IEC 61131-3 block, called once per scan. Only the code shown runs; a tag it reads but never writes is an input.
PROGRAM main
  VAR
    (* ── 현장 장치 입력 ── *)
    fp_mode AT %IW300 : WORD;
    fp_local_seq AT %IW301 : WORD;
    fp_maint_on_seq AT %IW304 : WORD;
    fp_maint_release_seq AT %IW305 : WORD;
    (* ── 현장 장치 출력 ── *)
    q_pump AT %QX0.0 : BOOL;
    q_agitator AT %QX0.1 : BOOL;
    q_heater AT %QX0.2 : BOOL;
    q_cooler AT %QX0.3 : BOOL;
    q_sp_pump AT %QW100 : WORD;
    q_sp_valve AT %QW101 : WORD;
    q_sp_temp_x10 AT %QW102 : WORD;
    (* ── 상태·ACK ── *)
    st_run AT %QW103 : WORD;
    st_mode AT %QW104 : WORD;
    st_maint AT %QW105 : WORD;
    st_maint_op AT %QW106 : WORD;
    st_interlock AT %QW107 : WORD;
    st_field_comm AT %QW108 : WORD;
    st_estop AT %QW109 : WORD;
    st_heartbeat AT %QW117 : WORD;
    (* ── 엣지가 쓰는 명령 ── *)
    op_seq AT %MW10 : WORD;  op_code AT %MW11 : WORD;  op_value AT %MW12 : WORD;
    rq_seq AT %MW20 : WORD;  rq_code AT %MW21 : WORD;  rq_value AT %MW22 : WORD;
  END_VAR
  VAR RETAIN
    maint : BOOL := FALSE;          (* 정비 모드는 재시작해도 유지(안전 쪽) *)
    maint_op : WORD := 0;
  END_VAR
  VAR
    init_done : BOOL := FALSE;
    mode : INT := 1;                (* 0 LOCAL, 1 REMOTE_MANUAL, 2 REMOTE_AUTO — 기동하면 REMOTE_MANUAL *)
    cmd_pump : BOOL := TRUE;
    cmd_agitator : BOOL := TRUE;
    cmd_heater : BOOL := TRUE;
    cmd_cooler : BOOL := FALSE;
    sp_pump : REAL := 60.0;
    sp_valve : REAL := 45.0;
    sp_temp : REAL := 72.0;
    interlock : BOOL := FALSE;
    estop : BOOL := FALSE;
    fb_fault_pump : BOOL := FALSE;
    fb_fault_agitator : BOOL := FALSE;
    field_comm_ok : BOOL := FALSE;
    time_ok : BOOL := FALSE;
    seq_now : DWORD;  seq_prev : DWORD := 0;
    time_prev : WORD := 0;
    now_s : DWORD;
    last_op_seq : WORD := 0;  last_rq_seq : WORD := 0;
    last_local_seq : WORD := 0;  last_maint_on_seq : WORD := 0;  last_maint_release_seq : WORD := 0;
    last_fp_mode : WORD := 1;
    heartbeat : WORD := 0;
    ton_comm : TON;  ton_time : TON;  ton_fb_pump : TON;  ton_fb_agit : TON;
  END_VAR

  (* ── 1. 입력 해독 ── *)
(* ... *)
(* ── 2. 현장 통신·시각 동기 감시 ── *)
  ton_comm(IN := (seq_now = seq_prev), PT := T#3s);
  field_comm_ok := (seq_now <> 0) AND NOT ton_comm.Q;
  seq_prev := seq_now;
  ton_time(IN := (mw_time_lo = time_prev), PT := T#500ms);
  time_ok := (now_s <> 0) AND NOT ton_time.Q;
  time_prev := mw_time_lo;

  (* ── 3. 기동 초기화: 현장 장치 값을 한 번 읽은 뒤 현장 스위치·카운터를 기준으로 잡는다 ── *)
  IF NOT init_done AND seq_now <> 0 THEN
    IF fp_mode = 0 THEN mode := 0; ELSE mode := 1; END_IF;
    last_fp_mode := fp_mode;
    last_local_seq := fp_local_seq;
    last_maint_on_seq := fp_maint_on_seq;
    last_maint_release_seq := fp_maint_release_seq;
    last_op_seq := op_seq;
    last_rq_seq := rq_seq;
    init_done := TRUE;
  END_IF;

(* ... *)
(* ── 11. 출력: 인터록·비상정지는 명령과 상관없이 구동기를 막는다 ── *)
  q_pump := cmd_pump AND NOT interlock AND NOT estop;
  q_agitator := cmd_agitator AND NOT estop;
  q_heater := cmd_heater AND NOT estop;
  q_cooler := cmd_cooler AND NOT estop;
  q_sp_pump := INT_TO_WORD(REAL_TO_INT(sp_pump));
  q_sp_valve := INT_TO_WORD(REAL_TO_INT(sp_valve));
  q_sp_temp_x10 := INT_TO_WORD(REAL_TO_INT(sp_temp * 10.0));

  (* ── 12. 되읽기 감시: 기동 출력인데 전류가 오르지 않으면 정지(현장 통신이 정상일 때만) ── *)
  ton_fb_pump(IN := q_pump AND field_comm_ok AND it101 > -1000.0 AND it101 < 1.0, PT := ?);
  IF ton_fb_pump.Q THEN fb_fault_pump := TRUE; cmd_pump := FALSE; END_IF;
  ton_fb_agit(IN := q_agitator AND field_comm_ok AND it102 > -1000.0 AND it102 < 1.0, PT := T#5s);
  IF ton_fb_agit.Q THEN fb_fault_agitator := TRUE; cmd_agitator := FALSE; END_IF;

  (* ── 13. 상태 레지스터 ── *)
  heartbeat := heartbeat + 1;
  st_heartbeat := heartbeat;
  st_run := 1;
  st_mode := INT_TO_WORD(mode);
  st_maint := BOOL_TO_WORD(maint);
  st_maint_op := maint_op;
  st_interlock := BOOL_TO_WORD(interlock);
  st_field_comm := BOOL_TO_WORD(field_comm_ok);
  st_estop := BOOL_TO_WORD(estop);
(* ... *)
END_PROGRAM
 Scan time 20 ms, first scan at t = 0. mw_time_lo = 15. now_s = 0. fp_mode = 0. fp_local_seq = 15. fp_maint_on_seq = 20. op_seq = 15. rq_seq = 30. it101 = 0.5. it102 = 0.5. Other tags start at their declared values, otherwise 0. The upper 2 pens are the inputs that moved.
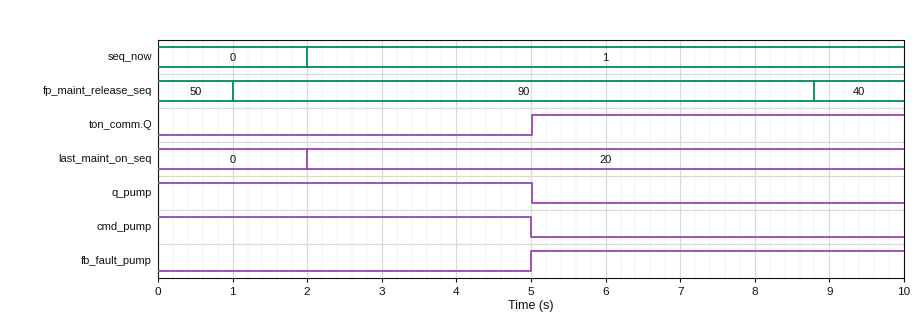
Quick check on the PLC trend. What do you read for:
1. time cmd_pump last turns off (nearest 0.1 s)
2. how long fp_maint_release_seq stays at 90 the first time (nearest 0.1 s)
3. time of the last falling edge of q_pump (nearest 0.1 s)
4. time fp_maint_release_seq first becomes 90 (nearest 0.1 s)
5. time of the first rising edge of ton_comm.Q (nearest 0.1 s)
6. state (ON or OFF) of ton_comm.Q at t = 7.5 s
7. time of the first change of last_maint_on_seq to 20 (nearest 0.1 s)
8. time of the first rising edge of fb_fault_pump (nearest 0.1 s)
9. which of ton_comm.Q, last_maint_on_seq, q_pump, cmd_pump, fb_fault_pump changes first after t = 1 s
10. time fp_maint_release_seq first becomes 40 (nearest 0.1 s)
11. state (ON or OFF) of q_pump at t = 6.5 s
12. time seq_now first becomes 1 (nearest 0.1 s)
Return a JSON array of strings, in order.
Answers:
["5.0 s", "7.8 s", "5.0 s", "1.0 s", "5.0 s", "ON", "2.0 s", "5.0 s", "last_maint_on_seq", "8.8 s", "OFF", "2.0 s"]
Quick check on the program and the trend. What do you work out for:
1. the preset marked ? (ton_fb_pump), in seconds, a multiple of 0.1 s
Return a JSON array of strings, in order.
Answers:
["3.0 s"]
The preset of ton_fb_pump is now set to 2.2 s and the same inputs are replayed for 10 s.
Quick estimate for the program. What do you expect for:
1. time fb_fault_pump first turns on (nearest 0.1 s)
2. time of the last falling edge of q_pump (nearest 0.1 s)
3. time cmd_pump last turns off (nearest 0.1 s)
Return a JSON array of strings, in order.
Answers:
["4.2 s", "4.2 s", "4.2 s"]
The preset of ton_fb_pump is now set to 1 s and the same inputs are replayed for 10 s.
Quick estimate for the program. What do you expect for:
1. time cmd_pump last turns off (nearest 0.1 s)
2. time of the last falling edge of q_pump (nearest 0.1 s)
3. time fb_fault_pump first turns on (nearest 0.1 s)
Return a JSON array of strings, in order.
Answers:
["3.0 s", "3.0 s", "3.0 s"]
